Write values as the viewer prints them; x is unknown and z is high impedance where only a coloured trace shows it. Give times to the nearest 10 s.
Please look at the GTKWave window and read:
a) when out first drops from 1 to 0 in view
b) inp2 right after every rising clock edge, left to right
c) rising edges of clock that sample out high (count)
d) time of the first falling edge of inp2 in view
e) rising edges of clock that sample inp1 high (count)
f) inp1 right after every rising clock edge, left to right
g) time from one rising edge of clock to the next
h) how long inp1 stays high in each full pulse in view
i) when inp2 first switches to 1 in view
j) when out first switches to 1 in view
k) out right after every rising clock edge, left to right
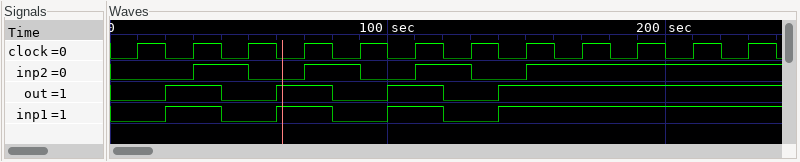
40 s
0 1 0 1 0 1 0 1 1 1 1 1
8
50 s
8
0 1 0 1 0 1 0 1 1 1 1 1
20 s
20 s, 20 s, 20 s
30 s
20 s
0 1 0 1 0 1 0 1 1 1 1 1
